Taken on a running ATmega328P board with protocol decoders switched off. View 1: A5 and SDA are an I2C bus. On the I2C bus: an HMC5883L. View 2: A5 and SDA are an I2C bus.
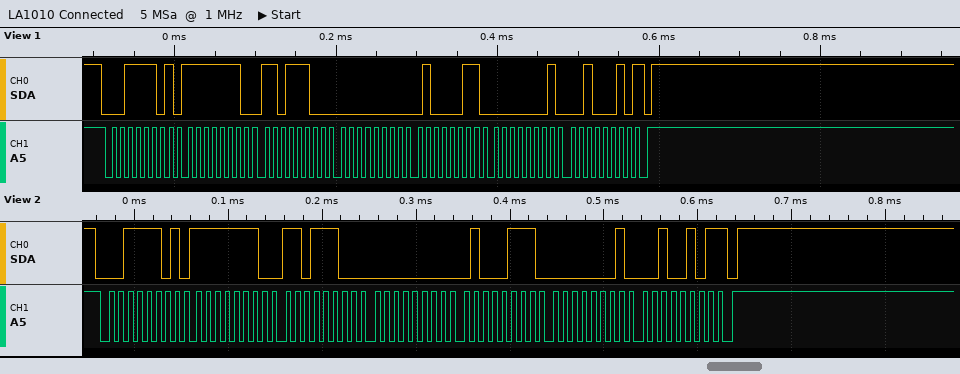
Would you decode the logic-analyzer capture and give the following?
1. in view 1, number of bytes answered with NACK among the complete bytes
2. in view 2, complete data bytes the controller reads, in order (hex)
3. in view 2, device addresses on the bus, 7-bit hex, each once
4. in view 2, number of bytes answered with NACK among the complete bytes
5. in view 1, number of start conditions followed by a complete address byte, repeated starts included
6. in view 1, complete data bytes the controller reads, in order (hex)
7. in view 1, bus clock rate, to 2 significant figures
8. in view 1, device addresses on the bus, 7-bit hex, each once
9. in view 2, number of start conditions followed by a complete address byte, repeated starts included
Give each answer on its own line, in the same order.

1
FE DC 00 47 01 25
0x1E
1
1
FE DC 00 43 01 22
100 kHz
0x1E
1
